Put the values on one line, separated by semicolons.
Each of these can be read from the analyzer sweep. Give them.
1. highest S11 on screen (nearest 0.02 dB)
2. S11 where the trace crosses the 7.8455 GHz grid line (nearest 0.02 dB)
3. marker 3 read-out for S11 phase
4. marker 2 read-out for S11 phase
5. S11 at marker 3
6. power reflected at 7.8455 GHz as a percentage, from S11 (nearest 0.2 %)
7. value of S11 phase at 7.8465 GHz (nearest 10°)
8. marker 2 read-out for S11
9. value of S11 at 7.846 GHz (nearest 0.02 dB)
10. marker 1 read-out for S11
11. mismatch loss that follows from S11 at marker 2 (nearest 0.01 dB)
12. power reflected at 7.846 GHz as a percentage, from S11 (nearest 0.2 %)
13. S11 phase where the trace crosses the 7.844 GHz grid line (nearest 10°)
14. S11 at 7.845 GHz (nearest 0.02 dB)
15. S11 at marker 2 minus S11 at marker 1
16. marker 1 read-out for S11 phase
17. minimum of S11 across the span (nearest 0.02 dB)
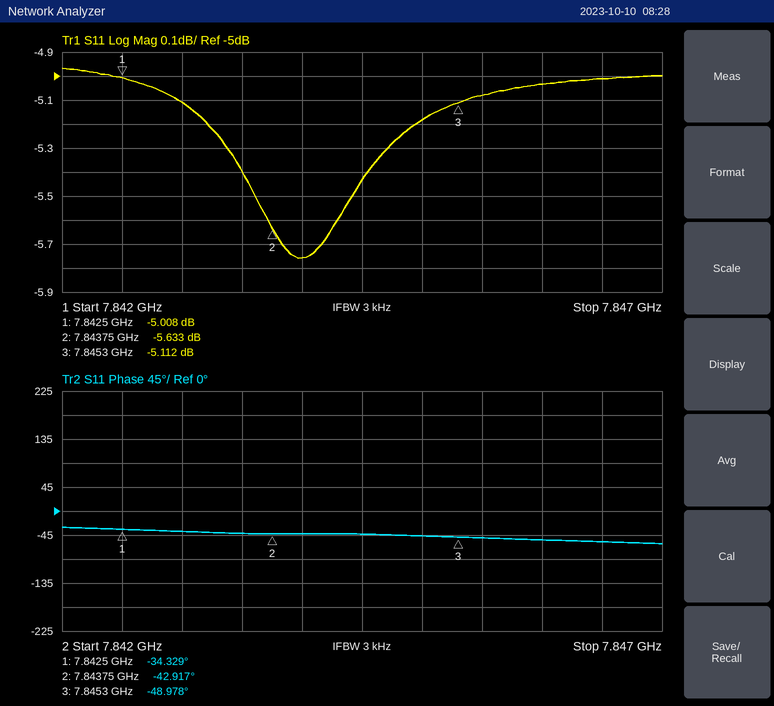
-4.96 dB; -5.08 dB; -48.978°; -42.917°; -5.112 dB; 31.0 %; -60°; -5.633 dB; -5.04 dB; -5.008 dB; 1.39 dB; 31.4 %; -40°; -5.18 dB; -0.625 dB; -34.329°; -5.76 dB
